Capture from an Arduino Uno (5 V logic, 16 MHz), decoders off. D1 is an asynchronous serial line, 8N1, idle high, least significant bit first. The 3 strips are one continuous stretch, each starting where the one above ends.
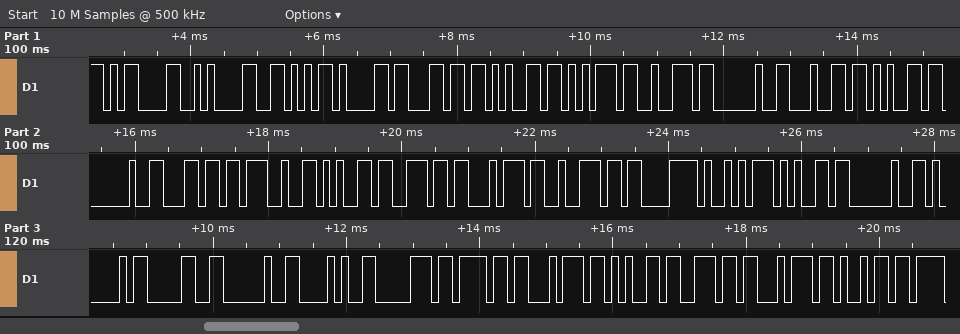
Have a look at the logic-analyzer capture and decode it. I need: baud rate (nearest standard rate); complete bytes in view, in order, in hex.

9600 baud
0D 0A 56 61 6C 65 75 72 20 64 65 20 6C 27 65 6E 74 72 C3 A9 65 20 41 30 20 28 70 6F 74 65 6E 74 69
